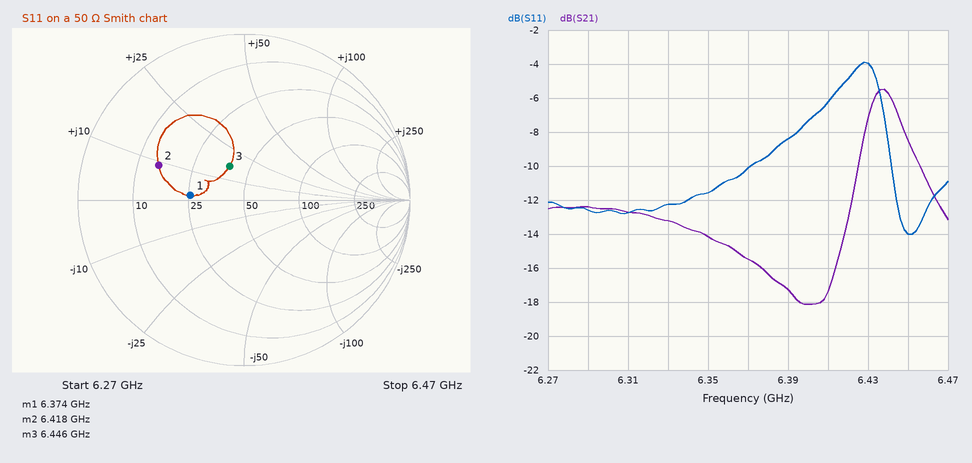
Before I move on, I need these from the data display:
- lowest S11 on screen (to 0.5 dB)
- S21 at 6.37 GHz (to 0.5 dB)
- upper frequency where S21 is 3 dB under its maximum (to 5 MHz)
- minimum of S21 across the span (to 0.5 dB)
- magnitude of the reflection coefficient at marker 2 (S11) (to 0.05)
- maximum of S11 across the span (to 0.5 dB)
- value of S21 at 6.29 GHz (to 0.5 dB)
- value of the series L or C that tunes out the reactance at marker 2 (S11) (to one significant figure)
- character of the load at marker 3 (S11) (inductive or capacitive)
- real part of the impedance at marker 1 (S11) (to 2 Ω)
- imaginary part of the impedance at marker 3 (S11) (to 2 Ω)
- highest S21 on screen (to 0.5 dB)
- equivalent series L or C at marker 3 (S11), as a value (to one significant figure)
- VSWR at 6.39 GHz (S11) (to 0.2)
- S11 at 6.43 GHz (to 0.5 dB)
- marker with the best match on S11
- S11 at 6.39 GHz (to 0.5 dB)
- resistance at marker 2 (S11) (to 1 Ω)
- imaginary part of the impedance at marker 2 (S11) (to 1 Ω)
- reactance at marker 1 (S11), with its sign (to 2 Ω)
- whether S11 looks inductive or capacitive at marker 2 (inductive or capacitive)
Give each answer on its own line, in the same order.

-14.0 dB
-15.5 dB
6.450 GHz
-18.0 dB
0.55
-4.0 dB
-12.5 dB
3 pF
inductive
26 Ω
+16 Ω
-5.5 dB
400 pH
2.2
-4.0 dB
marker 3
-8.5 dB
15 Ω
+9 Ω
+2 Ω
inductive
